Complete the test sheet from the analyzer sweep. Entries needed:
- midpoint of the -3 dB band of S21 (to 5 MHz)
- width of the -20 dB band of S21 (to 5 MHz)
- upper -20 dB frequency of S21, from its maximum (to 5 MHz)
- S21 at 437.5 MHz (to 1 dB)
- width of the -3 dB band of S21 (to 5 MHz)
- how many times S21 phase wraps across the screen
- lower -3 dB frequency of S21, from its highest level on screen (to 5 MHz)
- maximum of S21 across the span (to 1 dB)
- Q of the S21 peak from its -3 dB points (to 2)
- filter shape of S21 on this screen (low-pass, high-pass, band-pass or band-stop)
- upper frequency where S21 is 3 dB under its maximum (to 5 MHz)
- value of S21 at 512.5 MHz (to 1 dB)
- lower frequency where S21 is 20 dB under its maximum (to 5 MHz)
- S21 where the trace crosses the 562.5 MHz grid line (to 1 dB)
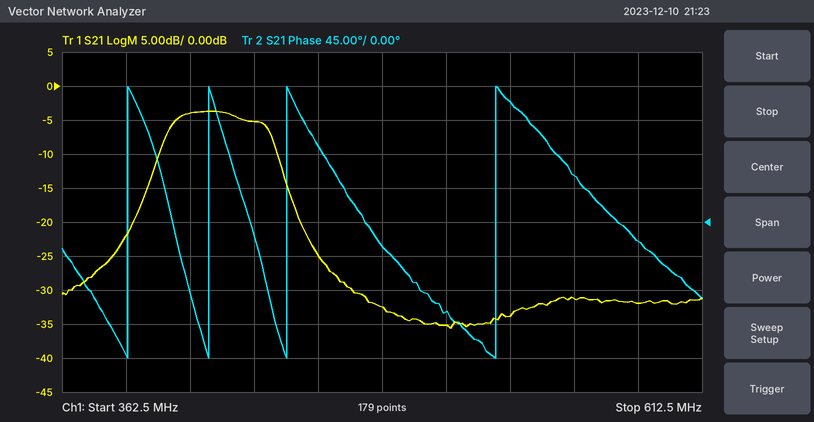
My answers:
425 MHz
75 MHz
460 MHz
-5 dB
40 MHz
4
405 MHz
-4 dB
10
band-pass
445 MHz
-35 dB
385 MHz
-31 dB
